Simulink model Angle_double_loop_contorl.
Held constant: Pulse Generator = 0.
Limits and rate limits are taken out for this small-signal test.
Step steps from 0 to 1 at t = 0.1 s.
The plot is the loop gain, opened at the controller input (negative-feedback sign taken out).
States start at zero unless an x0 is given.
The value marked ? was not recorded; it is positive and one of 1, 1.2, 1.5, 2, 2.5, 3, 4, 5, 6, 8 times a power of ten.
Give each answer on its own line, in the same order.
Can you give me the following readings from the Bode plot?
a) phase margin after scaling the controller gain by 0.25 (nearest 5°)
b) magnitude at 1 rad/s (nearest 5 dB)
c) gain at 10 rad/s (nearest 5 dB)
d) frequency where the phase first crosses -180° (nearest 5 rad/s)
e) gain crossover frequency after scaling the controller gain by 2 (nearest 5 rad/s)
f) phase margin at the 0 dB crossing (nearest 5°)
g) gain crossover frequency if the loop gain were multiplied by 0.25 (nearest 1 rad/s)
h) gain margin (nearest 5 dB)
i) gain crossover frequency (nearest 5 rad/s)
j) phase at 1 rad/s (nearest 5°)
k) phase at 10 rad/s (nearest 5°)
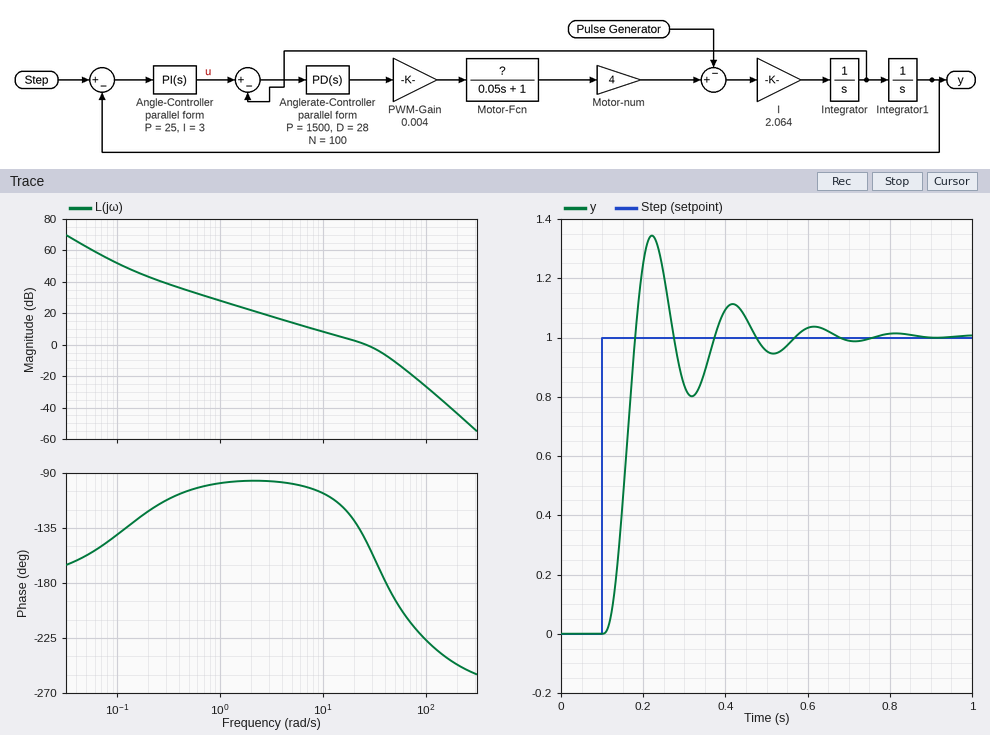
80°
30 dB
10 dB
40 rad/s
40 rad/s
35°
6 rad/s
5 dB
25 rad/s
-100°
-105°
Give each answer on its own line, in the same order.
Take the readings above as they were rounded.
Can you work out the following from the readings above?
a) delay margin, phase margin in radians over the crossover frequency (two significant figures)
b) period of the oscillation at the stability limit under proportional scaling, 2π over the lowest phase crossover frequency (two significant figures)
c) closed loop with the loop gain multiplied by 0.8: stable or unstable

0.024 s
0.16 s
stable
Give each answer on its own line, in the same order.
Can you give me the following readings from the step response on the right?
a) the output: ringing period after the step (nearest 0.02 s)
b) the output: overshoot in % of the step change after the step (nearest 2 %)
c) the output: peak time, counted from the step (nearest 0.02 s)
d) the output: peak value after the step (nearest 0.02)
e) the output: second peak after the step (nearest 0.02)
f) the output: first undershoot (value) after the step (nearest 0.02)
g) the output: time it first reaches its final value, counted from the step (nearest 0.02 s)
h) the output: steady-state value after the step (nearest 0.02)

0.20 s
34 %
0.12 s
1.34
1.12
0.80
0.08 s
1.00
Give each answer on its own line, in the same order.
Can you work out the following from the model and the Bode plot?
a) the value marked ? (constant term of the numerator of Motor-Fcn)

0.8
